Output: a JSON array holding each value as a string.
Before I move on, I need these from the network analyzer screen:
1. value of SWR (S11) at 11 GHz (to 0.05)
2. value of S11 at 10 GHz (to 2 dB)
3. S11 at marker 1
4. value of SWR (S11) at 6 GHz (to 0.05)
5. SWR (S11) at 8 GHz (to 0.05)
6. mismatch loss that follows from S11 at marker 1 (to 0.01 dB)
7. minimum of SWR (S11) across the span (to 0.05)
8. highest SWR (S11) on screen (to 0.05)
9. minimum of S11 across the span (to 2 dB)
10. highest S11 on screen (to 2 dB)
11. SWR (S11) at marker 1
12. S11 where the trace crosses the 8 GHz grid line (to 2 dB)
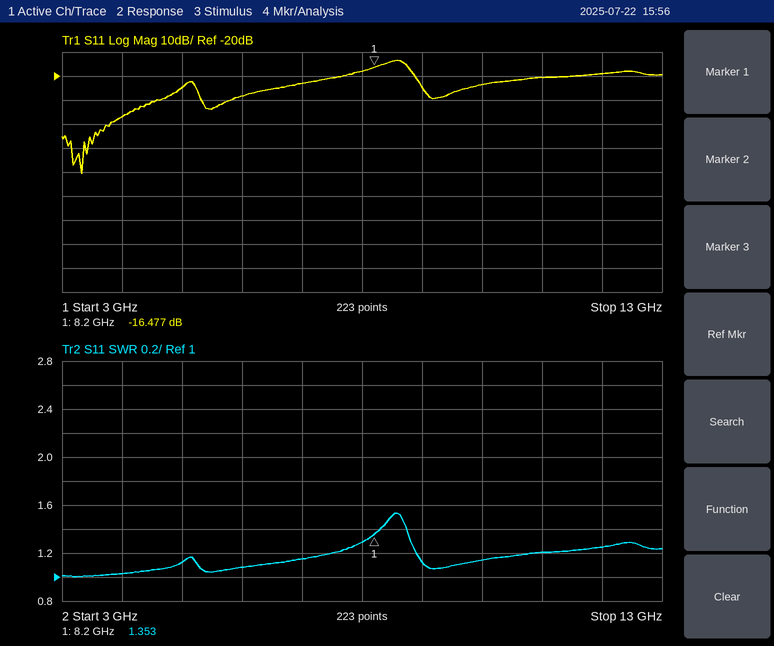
["1.20", "-24 dB", "-16.477 dB", "1.10", "1.30", "0.10 dB", "1.00", "1.55", "-60 dB", "-14 dB", "1.353", "-18 dB"]
